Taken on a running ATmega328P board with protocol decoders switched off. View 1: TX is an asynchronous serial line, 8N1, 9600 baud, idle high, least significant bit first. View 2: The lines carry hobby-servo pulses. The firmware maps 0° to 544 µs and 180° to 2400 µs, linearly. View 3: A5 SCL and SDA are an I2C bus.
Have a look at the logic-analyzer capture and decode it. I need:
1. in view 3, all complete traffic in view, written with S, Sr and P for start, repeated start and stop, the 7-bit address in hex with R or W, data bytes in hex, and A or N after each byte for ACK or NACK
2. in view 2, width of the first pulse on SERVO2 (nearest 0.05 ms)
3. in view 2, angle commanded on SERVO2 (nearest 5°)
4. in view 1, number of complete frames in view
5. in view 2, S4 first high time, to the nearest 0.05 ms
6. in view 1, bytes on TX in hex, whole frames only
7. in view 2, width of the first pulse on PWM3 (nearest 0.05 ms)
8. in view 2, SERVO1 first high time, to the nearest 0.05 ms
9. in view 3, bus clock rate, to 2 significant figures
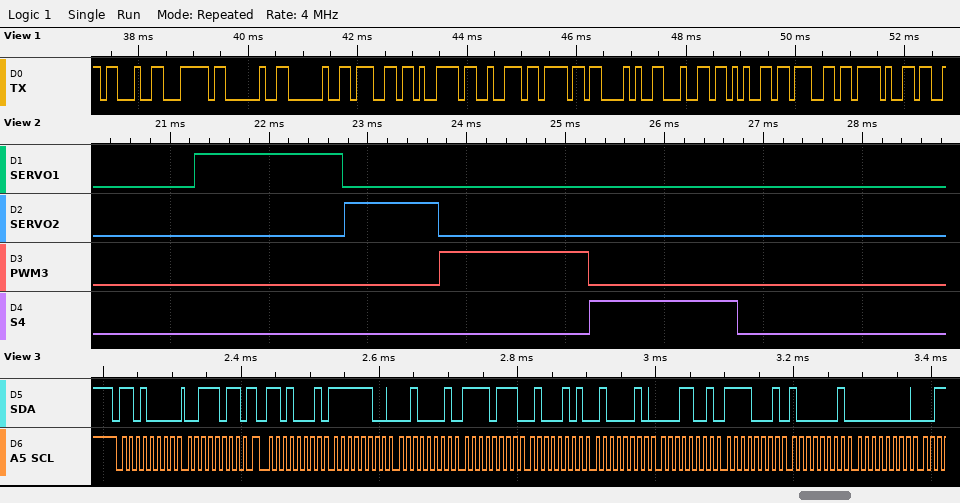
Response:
S 68W A 3B A Sr 68R A FC A 21 A F7 A 45 A 42 A 19 A F1 A 81 A 00 A
0.95 ms
40°
13
1.50 ms
23 7C 20 20 67 79 72 6F 28 64 65 67 2F
1.50 ms
1.50 ms
100 kHz
